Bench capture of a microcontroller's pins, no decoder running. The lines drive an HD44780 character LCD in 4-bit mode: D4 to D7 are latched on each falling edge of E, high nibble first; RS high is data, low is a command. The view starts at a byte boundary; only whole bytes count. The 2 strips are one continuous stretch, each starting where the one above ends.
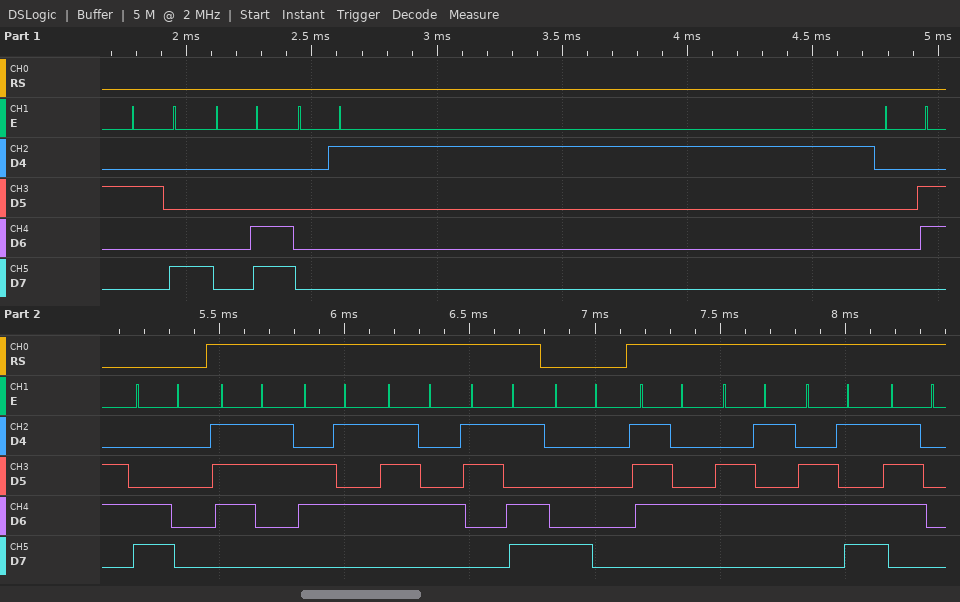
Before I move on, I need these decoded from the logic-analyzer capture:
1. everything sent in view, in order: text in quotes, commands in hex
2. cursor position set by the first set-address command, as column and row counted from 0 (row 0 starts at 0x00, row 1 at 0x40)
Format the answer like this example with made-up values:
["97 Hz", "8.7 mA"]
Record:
["0x28 0x0C 0x01 0x06 0xC0 \"set=\" 0x80 \"temp\"", "column 0, row 1"]
